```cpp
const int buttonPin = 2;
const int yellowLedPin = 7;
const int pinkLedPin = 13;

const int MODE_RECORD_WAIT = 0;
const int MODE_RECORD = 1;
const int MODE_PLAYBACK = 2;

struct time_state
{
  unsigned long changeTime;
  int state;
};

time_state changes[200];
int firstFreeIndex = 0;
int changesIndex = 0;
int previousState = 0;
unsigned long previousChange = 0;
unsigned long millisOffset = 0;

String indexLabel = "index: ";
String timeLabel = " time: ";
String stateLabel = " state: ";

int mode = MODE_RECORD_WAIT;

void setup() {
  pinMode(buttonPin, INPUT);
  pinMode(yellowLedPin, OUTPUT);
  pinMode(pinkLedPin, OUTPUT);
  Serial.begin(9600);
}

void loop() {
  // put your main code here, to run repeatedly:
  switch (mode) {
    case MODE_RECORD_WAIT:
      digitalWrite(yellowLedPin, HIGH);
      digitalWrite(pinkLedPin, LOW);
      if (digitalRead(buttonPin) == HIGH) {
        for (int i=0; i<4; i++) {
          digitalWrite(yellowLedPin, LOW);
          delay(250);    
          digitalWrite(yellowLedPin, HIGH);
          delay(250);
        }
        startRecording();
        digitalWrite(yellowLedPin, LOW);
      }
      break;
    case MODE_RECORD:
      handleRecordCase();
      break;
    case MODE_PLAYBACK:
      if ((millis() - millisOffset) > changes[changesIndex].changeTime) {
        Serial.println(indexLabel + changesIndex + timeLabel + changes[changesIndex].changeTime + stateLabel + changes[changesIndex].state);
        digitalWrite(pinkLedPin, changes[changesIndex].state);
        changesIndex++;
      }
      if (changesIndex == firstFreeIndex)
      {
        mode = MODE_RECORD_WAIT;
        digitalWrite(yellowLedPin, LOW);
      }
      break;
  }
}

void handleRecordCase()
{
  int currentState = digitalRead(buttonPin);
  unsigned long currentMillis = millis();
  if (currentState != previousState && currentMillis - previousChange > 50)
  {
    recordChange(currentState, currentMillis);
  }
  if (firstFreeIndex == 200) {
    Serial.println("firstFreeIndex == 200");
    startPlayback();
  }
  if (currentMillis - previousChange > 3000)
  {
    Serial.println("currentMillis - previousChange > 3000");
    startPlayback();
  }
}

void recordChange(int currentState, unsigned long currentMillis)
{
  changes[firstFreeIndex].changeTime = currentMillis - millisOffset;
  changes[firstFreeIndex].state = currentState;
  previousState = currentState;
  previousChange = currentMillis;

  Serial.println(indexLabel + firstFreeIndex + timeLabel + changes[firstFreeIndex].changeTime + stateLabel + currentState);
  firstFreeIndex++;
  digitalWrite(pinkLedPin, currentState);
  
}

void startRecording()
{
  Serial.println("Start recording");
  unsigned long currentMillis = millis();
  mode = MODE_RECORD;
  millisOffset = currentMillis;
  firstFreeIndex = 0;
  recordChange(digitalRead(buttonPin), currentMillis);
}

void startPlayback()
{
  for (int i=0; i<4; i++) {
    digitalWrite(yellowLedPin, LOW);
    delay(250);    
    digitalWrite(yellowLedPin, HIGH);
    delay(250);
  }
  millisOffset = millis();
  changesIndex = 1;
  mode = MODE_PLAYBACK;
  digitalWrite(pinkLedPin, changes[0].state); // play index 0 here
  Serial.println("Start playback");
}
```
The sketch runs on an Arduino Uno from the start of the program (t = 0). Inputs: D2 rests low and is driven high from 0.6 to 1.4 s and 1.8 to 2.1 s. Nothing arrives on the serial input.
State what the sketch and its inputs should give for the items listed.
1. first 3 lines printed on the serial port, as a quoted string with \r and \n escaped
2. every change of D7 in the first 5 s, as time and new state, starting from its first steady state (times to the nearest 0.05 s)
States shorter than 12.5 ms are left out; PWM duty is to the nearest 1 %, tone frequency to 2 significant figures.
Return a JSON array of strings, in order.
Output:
["\"Start recording\\r\\nindex: 0 time: 0 state: 0\\r\\ncurrentMillis - previousChange > 3000\\r\\n\"", "0 s high; 0.6 s low; 0.85 s high; 1.1 s low; 1.35 s high; 1.6 s low; 1.85 s high; 2.1 s low; 2.35 s high; 2.6 s low"]
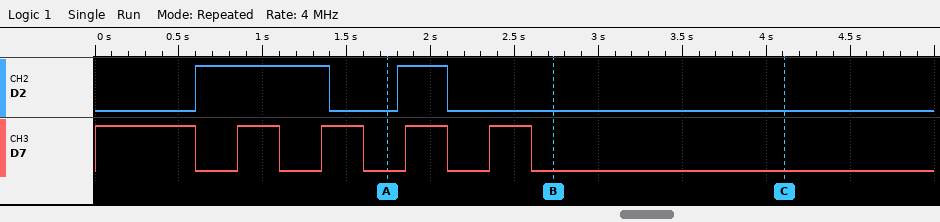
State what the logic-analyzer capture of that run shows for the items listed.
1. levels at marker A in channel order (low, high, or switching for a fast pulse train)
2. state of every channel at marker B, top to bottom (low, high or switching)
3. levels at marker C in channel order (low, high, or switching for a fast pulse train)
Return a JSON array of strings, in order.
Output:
["D2 low, D7 low", "D2 low, D7 low", "D2 low, D7 low"]
